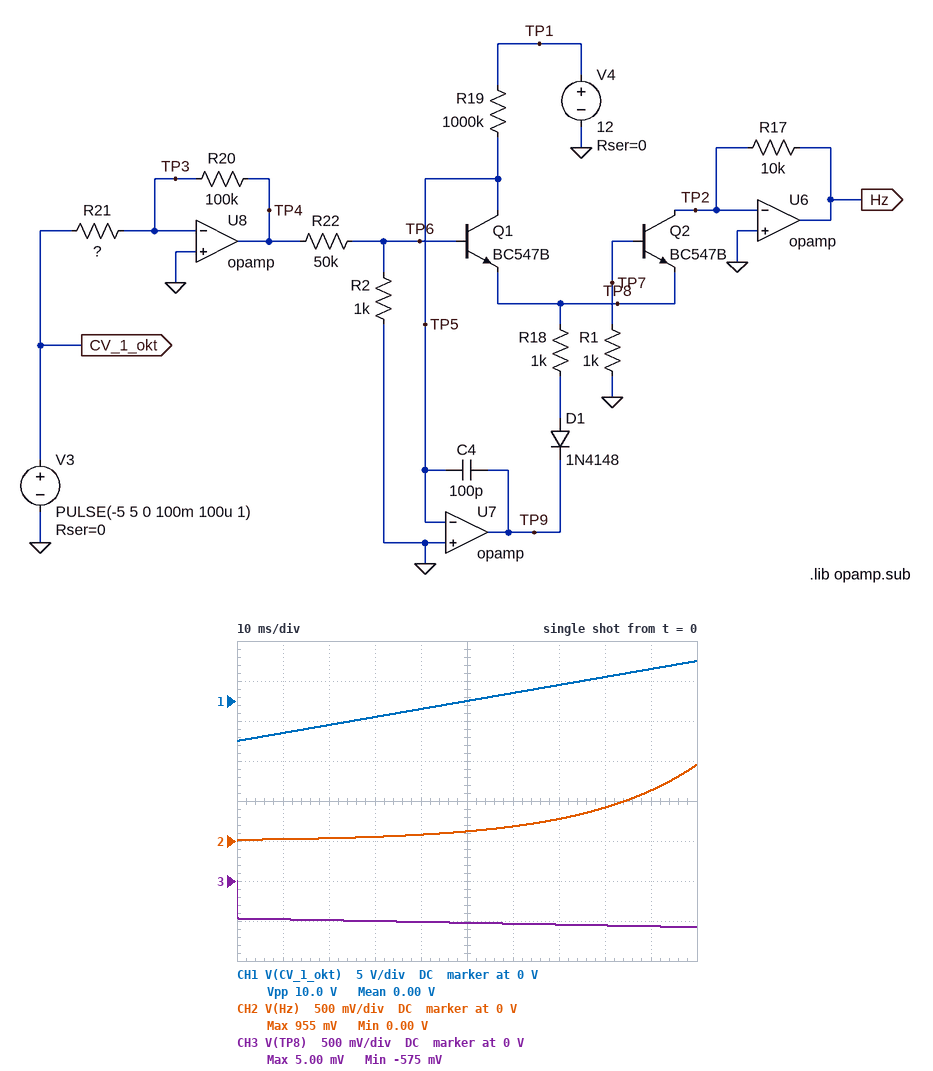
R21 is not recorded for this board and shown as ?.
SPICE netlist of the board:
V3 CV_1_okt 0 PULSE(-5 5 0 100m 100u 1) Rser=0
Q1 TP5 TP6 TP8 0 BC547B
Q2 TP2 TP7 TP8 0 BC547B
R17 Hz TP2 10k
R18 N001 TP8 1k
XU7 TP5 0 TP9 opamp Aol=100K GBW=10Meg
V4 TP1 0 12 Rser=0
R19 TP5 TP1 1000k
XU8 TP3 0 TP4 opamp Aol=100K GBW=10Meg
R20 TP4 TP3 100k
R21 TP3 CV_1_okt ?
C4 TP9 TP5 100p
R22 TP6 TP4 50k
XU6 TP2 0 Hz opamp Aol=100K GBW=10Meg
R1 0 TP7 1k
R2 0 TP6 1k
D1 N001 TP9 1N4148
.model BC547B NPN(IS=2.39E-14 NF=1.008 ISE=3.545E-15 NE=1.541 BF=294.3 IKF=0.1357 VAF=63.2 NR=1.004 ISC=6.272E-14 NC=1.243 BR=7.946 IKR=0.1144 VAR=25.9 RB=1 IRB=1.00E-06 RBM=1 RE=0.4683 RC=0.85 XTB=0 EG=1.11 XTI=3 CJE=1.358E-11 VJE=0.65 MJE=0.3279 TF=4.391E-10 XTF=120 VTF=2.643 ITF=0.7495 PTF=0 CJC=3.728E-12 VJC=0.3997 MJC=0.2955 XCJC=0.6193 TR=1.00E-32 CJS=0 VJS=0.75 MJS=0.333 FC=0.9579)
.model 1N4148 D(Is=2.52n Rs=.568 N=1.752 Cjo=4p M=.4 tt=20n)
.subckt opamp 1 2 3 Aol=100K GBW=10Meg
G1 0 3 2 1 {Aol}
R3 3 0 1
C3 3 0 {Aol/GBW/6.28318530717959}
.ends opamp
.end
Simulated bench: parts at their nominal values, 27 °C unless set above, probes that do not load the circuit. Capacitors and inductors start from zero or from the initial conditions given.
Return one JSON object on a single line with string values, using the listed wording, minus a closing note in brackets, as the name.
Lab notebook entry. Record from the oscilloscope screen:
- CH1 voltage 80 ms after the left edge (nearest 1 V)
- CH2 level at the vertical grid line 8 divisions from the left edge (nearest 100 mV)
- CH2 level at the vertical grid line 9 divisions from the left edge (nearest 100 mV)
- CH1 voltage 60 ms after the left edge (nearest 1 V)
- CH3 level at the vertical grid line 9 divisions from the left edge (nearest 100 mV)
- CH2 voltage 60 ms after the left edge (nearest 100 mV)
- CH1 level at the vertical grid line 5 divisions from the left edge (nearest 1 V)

{"CH1 voltage 80 ms after the left edge": "3 V", "CH2 level at the vertical grid line 8 divisions from the left edge": "400 mV", "CH2 level at the vertical grid line 9 divisions from the left edge": "600 mV", "CH1 voltage 60 ms after the left edge": "1 V", "CH3 level at the vertical grid line 9 divisions from the left edge": "-600 mV", "CH2 voltage 60 ms after the left edge": "200 mV", "CH1 level at the vertical grid line 5 divisions from the left edge": "0 V"}
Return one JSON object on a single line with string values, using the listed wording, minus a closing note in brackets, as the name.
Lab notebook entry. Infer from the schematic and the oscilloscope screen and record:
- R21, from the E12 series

{"R21, from the E12 series": "180 kΩ"}
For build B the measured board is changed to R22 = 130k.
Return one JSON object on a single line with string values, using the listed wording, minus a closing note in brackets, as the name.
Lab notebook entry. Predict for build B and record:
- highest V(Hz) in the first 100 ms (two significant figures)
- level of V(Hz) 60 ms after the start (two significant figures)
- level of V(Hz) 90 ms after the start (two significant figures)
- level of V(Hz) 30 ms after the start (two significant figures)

{"highest V(Hz) in the first 100 ms": "270 mV", "level of V(Hz) 60 ms after the start": "140 mV", "level of V(Hz) 90 ms after the start": "230 mV", "level of V(Hz) 30 ms after the start": "87 mV"}
